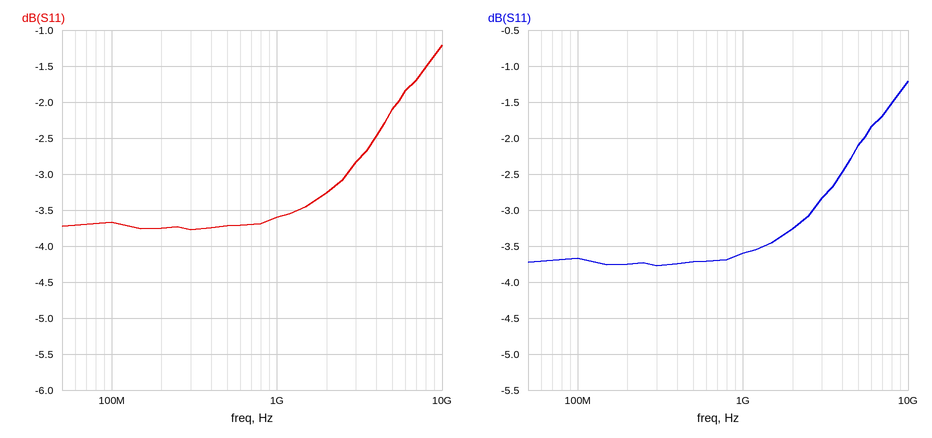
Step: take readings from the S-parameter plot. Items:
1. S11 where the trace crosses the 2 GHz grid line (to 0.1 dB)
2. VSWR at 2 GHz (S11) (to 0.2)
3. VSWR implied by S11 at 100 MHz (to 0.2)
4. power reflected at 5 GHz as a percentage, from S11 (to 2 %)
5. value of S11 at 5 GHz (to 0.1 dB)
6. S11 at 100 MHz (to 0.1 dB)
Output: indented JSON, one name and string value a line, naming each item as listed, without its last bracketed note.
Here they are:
{
  "S11 where the trace crosses the 2 GHz grid line": "-3.3 dB",
  "VSWR at 2 GHz (S11)": "5.4",
  "VSWR implied by S11 at 100 MHz": "4.8",
  "power reflected at 5 GHz as a percentage, from S11": "62 %",
  "value of S11 at 5 GHz": "-2.1 dB",
  "S11 at 100 MHz": "-3.7 dB"
}
